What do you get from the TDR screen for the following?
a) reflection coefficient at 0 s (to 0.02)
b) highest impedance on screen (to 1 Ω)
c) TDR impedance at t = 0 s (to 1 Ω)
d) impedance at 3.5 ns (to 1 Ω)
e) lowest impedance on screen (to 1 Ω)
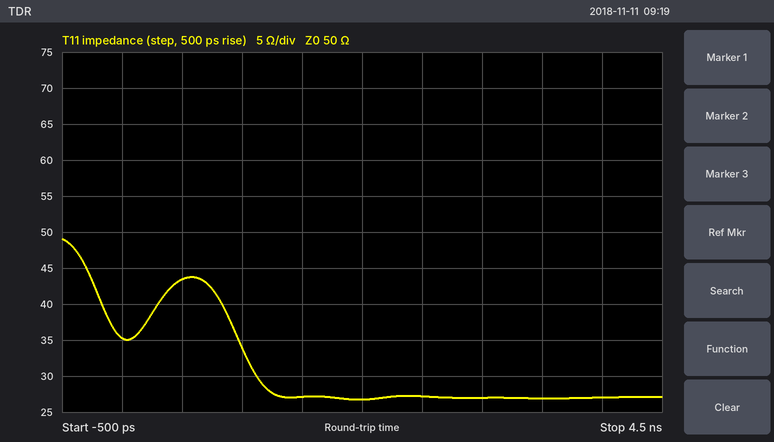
-0.18
49 Ω
35 Ω
27 Ω
27 Ω
